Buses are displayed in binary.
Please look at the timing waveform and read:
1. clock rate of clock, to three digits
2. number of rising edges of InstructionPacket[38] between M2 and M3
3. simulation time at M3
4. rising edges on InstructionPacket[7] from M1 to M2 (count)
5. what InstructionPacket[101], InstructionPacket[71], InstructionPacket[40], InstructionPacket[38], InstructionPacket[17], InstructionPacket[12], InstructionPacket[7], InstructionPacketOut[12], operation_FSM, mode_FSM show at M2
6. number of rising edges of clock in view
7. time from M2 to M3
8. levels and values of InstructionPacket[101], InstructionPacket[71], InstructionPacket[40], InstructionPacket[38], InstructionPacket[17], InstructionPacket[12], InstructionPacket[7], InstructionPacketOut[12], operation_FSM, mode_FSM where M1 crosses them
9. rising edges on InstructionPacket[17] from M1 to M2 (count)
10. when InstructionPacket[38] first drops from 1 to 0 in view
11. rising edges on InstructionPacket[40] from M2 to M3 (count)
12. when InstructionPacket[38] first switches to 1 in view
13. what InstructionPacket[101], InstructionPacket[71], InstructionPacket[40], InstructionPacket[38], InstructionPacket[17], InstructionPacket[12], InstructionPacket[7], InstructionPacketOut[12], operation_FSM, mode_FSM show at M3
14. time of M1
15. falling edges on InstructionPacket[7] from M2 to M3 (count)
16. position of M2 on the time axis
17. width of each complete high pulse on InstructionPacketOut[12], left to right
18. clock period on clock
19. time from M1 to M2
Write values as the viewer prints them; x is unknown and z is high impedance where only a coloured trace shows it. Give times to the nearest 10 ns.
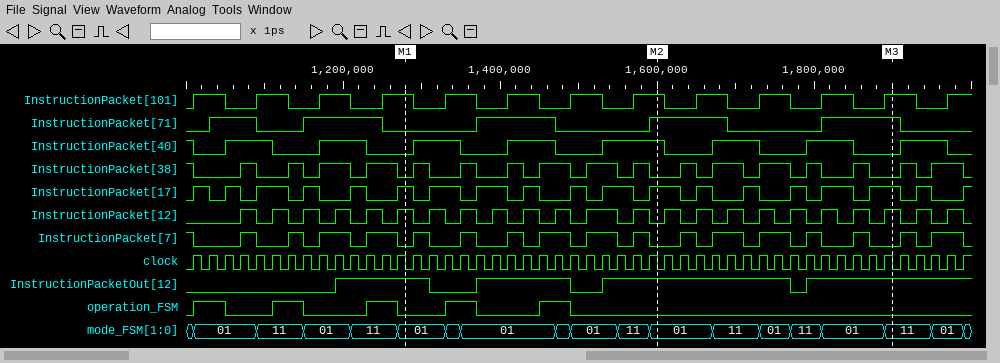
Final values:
50.0 MHz
5
1900 ns
6
InstructionPacket[101]=1, InstructionPacket[71]=1, InstructionPacket[40]=1, InstructionPacket[38]=0, InstructionPacket[17]=1, InstructionPacket[12]=0, InstructionPacket[7]=0, InstructionPacketOut[12]=1, operation_FSM=0, mode_FSM=01
50
300 ns
InstructionPacket[101]=1, InstructionPacket[71]=0, InstructionPacket[40]=0, InstructionPacket[38]=0, InstructionPacket[17]=1, InstructionPacket[12]=1, InstructionPacket[7]=0, InstructionPacketOut[12]=1, operation_FSM=0, mode_FSM=01
6
1010 ns
2
1070 ns
InstructionPacket[101]=1, InstructionPacket[71]=1, InstructionPacket[40]=0, InstructionPacket[38]=0, InstructionPacket[17]=1, InstructionPacket[12]=1, InstructionPacket[7]=0, InstructionPacketOut[12]=1, operation_FSM=0, mode_FSM=11
1280 ns
5
1600 ns
120 ns, 120 ns, 240 ns
20 ns
320 ns
